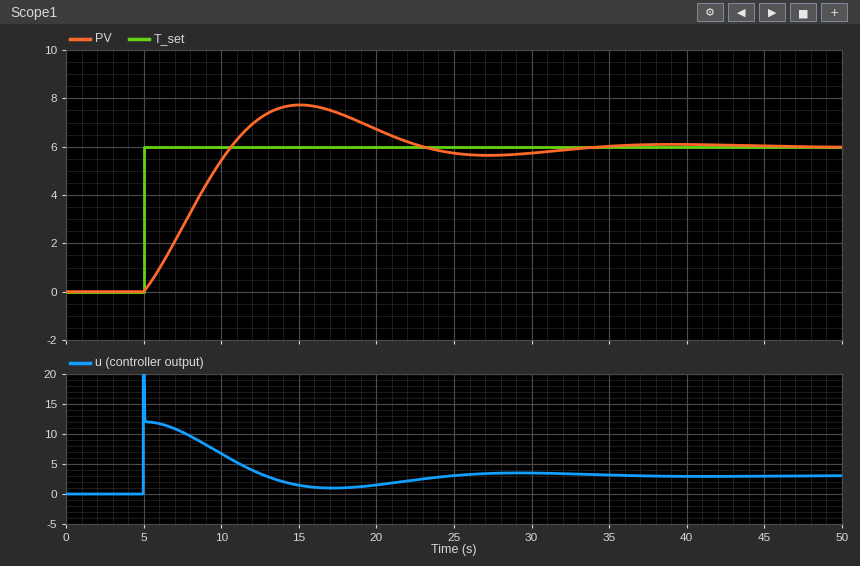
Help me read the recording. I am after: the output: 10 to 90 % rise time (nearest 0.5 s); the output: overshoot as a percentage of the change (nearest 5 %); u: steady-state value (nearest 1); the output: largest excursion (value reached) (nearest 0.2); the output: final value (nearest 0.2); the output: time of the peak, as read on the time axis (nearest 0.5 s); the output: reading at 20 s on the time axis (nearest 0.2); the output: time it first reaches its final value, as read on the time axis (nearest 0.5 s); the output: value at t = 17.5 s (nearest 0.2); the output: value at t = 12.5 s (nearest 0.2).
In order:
4.5 s
30 %
3
7.8
6.0
15.0 s
6.8
10.5 s
7.4
7.2
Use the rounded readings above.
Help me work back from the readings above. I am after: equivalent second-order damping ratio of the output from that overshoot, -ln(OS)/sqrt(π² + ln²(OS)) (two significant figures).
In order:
0.36
